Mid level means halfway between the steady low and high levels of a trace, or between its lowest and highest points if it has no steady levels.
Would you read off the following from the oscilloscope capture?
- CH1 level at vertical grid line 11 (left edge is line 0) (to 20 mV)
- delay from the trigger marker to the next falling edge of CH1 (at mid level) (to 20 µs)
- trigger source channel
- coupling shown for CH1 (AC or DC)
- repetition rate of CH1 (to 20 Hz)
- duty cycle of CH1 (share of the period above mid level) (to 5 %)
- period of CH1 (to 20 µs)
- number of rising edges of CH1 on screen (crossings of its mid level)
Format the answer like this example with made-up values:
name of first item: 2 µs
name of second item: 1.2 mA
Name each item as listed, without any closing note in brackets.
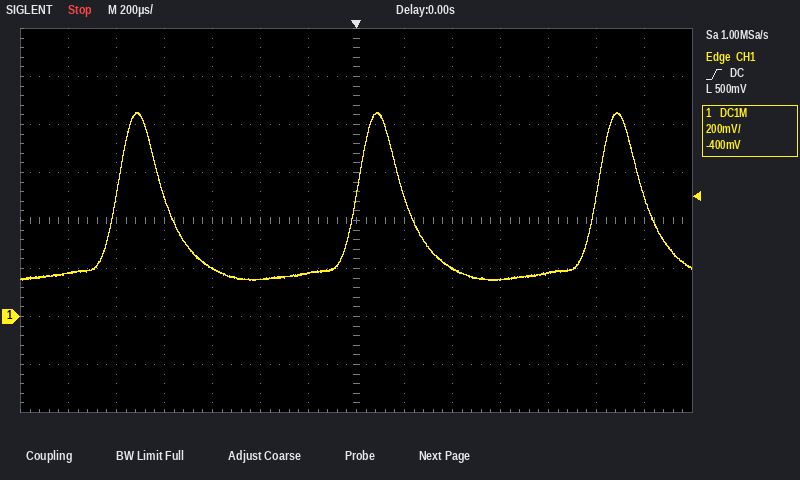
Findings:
CH1 level at vertical grid line 11 (left edge is line 0): 180 mV
delay from the trigger marker to the next falling edge of CH1 (at mid level): 200 µs
trigger source channel: CH1
coupling shown for CH1: DC
repetition rate of CH1: 1.00 kHz
duty cycle of CH1 (share of the period above mid level): 20 %
period of CH1: 1.00 ms
number of rising edges of CH1 on screen: 3
